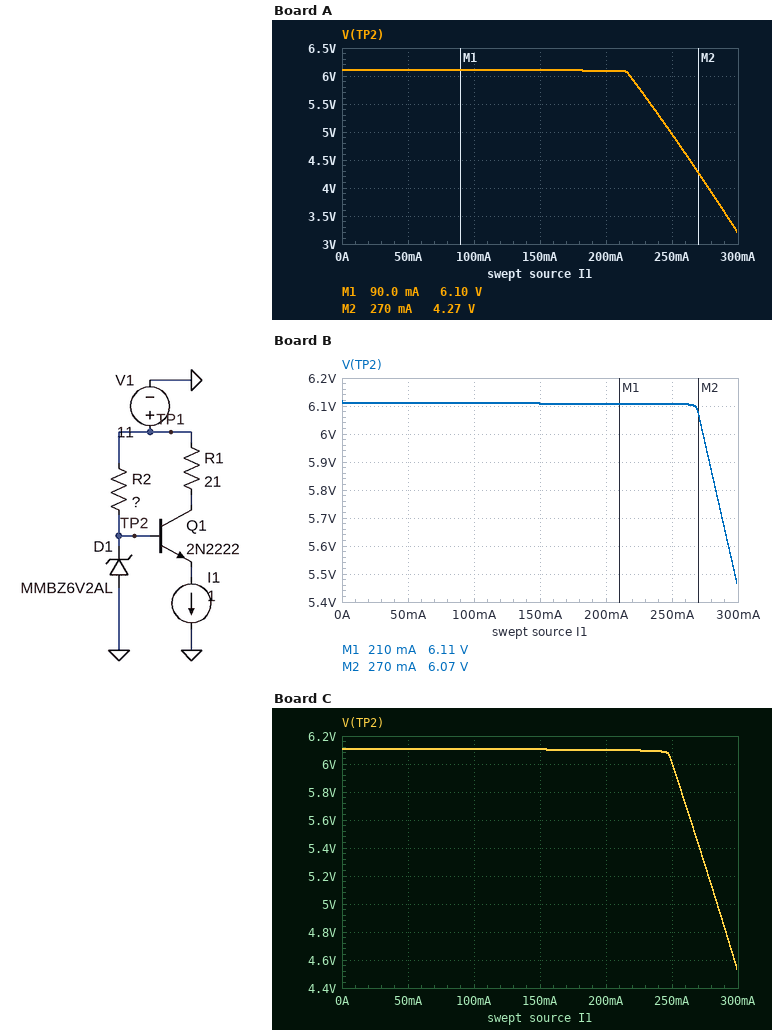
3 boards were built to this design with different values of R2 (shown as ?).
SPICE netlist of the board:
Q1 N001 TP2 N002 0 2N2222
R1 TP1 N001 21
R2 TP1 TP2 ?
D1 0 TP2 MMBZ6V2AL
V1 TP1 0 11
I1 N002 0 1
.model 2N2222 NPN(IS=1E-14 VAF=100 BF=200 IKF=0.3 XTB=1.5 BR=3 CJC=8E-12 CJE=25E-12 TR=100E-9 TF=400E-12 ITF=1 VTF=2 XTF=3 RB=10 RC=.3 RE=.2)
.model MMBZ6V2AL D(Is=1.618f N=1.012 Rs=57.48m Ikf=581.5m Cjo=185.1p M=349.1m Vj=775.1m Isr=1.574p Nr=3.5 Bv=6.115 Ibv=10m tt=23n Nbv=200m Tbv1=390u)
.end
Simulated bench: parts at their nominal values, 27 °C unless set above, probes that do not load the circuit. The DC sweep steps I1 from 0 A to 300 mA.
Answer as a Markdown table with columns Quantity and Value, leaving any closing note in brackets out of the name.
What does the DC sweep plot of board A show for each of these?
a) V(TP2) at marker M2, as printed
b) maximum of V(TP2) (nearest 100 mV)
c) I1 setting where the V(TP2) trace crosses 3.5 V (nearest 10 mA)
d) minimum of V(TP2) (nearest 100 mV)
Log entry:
| Quantity | Value |
|---|---|
| V(TP2) at marker M2, as printed | 4.27 V |
| maximum of V(TP2) | 6.1 V |
| I1 setting where the V(TP2) trace crosses 3.5 V | 290 mA |
| minimum of V(TP2) | 3.2 V |
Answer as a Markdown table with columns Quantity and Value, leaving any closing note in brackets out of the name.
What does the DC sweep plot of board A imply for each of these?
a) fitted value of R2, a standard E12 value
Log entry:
| Quantity | Value |
|---|---|
| fitted value of R2, a standard E12 value | 2.7 kΩ |
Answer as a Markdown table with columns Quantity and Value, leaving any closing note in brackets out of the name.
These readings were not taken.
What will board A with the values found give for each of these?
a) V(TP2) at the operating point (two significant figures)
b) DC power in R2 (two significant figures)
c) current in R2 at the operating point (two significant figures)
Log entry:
| Quantity | Value |
|---|---|
| V(TP2) at the operating point | -890 mV |
| DC power in R2 | 52 mW |
| current in R2 at the operating point | 4.4 mA |
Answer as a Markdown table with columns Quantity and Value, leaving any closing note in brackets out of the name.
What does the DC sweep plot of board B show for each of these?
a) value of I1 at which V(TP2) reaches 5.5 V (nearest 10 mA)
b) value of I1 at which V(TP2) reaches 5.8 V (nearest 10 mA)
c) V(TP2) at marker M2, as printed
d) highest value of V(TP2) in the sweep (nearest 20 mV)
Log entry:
| Quantity | Value |
|---|---|
| value of I1 at which V(TP2) reaches 5.5 V | 300 mA |
| value of I1 at which V(TP2) reaches 5.8 V | 280 mA |
| V(TP2) at marker M2, as printed | 6.07 V |
| highest value of V(TP2) in the sweep | 6.12 V |
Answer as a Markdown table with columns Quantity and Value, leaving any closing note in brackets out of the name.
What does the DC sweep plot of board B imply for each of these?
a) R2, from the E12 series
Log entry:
| Quantity | Value |
|---|---|
| R2, from the E12 series | 1.2 kΩ |
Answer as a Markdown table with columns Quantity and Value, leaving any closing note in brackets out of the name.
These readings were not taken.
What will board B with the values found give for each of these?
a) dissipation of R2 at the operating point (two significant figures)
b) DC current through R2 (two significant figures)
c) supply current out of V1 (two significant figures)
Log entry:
| Quantity | Value |
|---|---|
| dissipation of R2 at the operating point | 120 mW |
| DC current through R2 | 9.9 mA |
| supply current out of V1 | 740 mA |
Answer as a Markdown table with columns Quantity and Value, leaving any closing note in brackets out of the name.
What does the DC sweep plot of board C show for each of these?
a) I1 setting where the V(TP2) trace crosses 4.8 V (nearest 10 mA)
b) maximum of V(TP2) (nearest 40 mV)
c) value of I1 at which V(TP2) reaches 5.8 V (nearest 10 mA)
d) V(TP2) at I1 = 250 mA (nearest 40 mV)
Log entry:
| Quantity | Value |
|---|---|
| I1 setting where the V(TP2) trace crosses 4.8 V | 290 mA |
| maximum of V(TP2) | 6.12 V |
| value of I1 at which V(TP2) reaches 5.8 V | 260 mA |
| V(TP2) at I1 = 250 mA | 6.00 V |
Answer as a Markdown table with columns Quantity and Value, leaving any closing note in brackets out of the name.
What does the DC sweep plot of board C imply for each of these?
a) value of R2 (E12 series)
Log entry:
| Quantity | Value |
|---|---|
| value of R2 | 2.2 kΩ |
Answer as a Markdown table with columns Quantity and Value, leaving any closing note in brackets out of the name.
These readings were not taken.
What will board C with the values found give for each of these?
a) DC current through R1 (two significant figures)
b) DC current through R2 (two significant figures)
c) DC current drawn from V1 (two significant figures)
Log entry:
| Quantity | Value |
|---|---|
| DC current through R1 | 730 mA |
| DC current through R2 | 5.4 mA |
| DC current drawn from V1 | 730 mA |
